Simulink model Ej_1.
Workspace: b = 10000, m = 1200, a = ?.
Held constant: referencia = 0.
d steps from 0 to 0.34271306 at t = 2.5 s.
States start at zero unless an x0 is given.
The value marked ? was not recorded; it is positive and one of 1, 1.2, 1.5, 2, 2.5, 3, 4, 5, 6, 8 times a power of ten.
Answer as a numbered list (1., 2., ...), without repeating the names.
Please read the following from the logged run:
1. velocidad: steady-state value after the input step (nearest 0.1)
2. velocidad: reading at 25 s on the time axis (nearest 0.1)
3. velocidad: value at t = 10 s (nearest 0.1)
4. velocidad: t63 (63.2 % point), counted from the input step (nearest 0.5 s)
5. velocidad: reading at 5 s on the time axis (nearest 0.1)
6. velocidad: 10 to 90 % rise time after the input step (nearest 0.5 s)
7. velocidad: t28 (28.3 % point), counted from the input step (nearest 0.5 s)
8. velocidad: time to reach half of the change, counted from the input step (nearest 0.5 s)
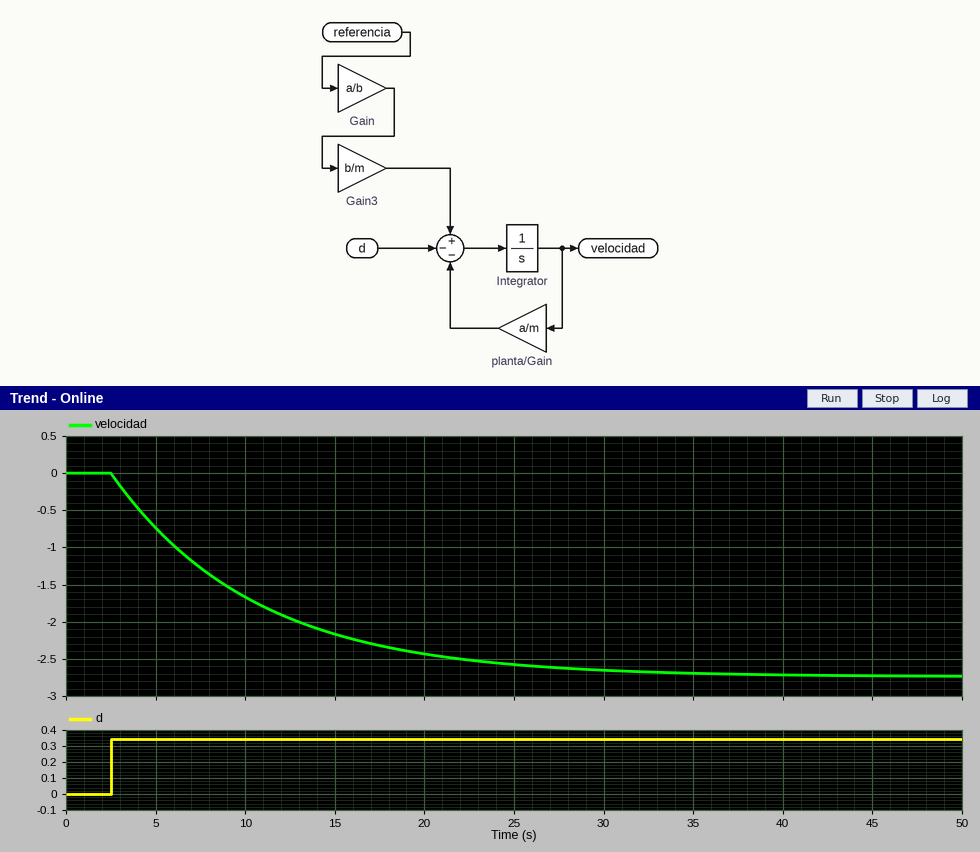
1. -2.7
2. -2.6
3. -1.7
4. 8.0 s
5. -0.7
6. 17.5 s
7. 2.5 s
8. 5.5 s
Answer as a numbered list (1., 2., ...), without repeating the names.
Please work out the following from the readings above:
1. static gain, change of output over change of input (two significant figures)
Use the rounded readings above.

1. -7.9
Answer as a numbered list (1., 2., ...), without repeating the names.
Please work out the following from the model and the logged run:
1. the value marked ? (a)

1. 150
